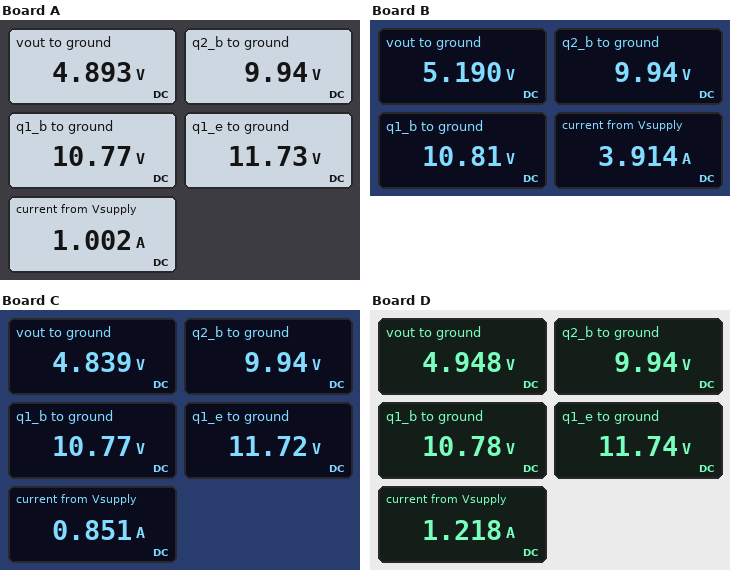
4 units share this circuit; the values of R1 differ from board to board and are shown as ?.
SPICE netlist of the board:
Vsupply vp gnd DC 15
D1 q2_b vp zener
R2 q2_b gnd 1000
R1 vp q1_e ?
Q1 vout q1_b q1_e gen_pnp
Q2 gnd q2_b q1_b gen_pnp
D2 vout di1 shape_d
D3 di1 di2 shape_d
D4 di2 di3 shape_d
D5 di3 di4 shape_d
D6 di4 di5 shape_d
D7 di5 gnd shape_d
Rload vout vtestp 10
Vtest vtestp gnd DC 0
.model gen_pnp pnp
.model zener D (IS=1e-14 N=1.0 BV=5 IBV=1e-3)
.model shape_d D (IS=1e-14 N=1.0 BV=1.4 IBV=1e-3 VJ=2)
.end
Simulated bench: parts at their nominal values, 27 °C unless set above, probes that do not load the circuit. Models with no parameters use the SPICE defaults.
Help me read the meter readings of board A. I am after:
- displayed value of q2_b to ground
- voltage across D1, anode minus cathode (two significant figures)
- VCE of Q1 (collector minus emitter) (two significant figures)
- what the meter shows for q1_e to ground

9.94 V
-5.1 V
-6.8 V
11.73 V
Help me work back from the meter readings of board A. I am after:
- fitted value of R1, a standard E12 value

3.3 Ω
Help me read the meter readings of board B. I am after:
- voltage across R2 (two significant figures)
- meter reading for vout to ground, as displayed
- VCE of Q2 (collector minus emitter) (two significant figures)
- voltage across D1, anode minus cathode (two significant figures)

9.9 V
5.190 V
-11 V
-5.1 V
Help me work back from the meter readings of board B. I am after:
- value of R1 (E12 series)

0.82 Ω
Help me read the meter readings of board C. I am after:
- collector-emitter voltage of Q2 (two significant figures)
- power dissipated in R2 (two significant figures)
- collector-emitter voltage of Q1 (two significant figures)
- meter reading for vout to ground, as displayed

-11 V
99 mW
-6.9 V
4.839 V
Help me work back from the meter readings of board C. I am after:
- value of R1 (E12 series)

3.9 Ω
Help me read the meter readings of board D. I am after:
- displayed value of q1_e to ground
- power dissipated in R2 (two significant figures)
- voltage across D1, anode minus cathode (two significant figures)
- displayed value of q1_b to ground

11.74 V
99 mW
-5.1 V
10.78 V
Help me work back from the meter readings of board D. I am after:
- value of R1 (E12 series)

2.7 Ω
